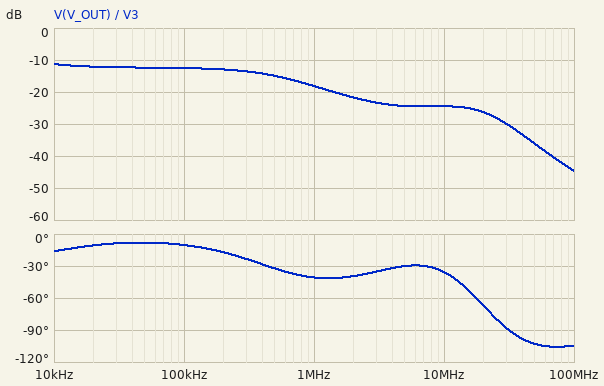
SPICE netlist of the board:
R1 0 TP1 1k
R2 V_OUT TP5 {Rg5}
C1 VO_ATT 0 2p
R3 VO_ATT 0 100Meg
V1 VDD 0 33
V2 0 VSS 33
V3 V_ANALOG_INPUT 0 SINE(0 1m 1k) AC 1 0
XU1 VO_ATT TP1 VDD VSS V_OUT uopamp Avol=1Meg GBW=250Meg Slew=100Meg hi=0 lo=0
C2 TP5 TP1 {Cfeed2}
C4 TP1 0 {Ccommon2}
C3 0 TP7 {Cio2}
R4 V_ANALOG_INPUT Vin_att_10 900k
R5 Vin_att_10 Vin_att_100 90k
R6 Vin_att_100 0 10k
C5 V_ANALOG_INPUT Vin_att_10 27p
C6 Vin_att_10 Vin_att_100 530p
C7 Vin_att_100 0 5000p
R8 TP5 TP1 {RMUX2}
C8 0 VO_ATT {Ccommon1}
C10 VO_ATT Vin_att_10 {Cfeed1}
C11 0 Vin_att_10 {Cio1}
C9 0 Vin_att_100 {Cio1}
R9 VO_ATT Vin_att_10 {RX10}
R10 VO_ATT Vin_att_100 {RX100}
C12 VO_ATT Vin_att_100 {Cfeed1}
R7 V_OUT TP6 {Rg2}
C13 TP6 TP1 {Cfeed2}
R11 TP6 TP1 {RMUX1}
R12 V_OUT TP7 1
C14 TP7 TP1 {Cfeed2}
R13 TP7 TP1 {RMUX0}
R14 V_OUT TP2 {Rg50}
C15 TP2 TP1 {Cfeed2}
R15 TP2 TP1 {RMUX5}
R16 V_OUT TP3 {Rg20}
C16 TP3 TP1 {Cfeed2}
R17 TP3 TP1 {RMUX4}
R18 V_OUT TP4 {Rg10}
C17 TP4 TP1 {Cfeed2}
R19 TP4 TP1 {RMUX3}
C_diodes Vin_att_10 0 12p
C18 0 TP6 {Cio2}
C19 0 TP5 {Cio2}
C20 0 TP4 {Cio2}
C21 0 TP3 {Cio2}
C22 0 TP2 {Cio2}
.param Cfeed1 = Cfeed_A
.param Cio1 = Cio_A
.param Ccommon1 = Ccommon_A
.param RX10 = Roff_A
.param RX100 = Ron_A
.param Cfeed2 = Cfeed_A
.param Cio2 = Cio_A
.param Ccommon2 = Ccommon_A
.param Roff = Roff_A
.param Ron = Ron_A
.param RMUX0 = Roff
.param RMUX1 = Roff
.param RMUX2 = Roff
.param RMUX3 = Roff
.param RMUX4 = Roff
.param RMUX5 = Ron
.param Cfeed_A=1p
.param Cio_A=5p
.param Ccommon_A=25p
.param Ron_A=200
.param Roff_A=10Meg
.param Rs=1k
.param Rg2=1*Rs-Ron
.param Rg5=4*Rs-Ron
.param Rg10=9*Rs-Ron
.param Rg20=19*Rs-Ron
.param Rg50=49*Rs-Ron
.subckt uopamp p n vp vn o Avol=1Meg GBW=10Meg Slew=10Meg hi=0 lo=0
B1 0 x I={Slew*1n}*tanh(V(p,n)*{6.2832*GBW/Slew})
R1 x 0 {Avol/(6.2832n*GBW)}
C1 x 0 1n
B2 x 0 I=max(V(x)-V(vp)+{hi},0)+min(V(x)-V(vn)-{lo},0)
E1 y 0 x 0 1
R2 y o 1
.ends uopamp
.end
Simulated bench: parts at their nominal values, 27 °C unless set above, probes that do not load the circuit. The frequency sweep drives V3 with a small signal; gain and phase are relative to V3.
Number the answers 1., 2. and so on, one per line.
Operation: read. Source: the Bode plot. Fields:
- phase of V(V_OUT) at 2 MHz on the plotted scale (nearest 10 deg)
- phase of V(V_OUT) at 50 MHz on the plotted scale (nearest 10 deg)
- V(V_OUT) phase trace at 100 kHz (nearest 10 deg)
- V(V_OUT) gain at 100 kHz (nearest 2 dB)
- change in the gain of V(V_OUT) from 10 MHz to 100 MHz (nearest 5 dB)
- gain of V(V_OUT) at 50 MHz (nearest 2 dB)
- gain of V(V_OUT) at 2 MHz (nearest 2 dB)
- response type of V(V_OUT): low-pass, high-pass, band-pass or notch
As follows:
1. -40 deg
2. -100 deg
3. -10 deg
4. -12 dB
5. -20 dB
6. -36 dB
7. -22 dB
8. low-pass
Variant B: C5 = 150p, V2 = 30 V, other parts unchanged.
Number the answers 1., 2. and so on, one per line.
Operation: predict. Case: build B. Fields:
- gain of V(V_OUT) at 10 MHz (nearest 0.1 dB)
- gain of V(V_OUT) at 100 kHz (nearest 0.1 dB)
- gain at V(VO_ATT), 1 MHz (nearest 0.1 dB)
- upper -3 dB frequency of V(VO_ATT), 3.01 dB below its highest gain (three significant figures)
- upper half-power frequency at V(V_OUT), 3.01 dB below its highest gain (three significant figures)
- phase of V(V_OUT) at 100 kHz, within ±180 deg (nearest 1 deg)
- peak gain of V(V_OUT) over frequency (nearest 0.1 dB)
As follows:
1. -11.4 dB
2. 0.5 dB
3. -33.1 dB
4. 33.3 MHz
5. 567 kHz
6. -8 deg
7. 0.6 dB
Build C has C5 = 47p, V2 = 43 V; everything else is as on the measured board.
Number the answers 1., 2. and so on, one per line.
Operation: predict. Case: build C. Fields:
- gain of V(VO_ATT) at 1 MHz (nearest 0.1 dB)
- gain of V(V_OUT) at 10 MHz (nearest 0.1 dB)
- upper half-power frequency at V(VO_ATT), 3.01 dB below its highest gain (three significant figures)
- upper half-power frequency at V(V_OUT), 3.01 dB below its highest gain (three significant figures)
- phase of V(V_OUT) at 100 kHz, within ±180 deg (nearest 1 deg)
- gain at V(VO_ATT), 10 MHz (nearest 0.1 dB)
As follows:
1. -41.7 dB
2. -20.0 dB
3. 18.6 MHz
4. 327 kHz
5. -9 deg
6. -42.1 dB
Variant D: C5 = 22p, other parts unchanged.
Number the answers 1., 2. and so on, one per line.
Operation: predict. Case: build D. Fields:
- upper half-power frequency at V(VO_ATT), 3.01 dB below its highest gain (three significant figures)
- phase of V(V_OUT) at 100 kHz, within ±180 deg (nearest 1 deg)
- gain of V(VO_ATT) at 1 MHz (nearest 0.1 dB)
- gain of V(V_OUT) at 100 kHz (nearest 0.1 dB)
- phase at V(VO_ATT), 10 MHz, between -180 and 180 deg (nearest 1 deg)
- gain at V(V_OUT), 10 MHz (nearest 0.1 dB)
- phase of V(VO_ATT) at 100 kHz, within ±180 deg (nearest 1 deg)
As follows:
1. 3.95 kHz
2. -11 deg
3. -47.9 dB
4. -14.2 dB
5. -12 deg
6. -26.2 dB
7. -3 deg
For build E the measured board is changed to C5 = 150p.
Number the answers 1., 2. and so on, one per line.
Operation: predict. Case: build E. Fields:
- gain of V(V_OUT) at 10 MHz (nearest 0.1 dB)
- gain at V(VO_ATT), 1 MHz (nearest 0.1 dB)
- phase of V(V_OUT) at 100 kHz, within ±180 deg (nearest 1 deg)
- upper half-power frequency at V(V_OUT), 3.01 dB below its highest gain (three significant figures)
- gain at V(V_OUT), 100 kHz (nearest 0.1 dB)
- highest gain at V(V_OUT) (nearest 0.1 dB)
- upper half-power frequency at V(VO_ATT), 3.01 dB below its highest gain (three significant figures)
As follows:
1. -11.4 dB
2. -33.1 dB
3. -8 deg
4. 567 kHz
5. 0.5 dB
6. 0.6 dB
7. 33.3 MHz
